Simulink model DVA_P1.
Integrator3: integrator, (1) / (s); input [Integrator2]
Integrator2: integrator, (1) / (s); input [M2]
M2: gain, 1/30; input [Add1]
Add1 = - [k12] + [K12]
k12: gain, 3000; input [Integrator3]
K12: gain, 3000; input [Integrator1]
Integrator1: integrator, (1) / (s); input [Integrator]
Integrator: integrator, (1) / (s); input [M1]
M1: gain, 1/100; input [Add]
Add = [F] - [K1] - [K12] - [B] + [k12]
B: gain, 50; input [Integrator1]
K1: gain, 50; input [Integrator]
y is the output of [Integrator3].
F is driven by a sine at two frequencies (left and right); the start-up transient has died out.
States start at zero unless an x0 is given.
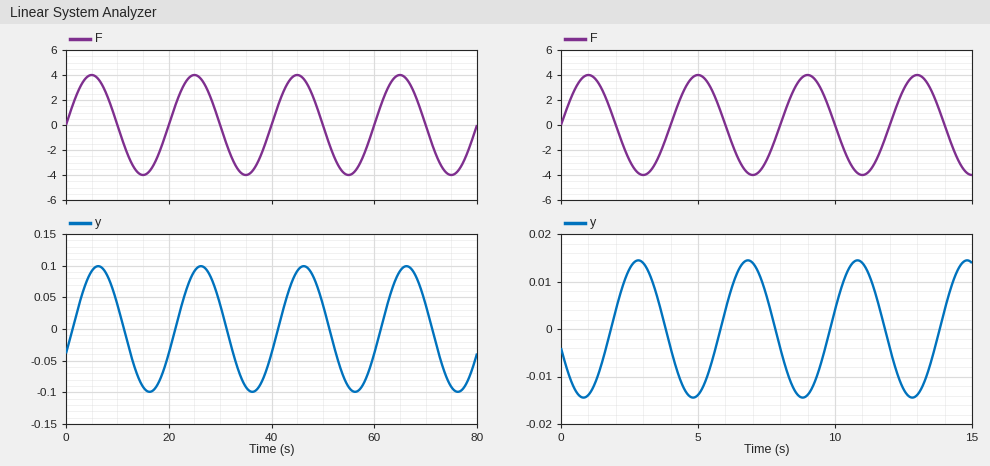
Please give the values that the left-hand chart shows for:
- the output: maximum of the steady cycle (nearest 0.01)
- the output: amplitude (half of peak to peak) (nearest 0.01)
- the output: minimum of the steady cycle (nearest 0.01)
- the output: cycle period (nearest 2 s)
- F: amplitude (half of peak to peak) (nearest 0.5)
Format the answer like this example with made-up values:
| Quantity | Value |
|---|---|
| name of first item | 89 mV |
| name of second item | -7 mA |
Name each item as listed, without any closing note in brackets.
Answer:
| Quantity | Value |
|---|---|
| the output: maximum of the steady cycle | 0.10 |
| the output: amplitude (half of peak to peak) | 0.10 |
| the output: minimum of the steady cycle | -0.10 |
| the output: cycle period | 20 s |
| F: amplitude (half of peak to peak) | 4.0 |
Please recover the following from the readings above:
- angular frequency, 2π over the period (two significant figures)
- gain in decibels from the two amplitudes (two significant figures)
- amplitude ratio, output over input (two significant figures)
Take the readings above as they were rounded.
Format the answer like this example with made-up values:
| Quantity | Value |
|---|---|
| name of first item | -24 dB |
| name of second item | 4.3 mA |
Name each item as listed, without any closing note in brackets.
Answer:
| Quantity | Value |
|---|---|
| angular frequency, 2π over the period | 0.31 rad/s |
| gain in decibels from the two amplitudes | -32 dB |
| amplitude ratio, output over input | 0.025 |
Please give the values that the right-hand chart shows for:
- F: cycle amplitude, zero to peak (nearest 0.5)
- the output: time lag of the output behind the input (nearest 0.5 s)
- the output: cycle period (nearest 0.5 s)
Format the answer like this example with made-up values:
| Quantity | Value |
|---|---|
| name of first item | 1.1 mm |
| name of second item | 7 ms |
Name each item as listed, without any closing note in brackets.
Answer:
| Quantity | Value |
|---|---|
| F: cycle amplitude, zero to peak | 4.0 |
| the output: time lag of the output behind the input | 2.0 s |
| the output: cycle period | 4.0 s |
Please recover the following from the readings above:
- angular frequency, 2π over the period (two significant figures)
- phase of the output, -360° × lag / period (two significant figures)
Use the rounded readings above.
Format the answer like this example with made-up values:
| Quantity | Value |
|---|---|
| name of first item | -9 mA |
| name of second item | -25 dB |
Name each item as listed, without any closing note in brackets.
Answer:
| Quantity | Value |
|---|---|
| angular frequency, 2π over the period | 1.6 rad/s |
| phase of the output, -360° × lag / period | -180° |
